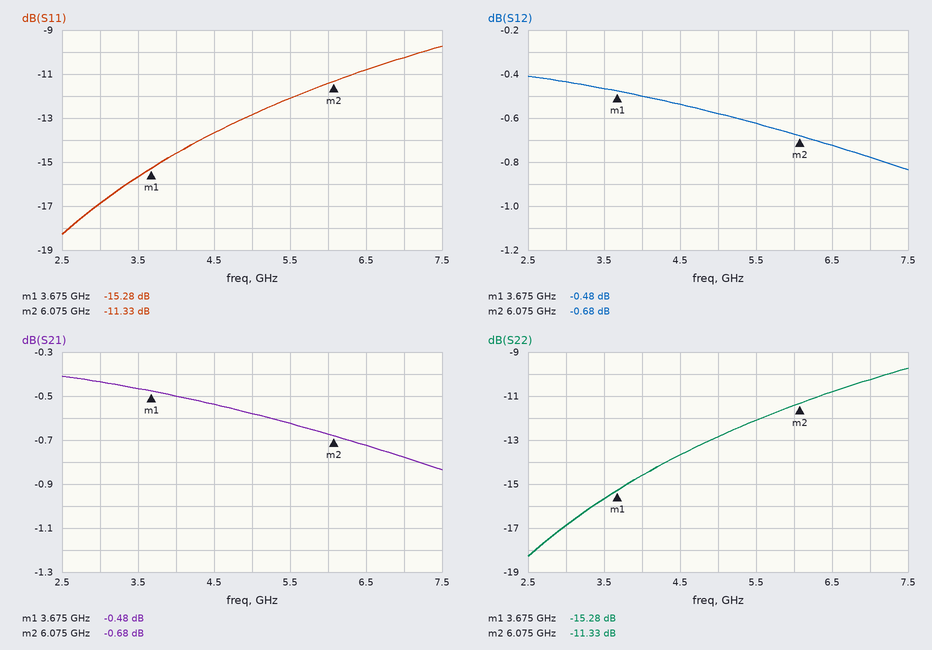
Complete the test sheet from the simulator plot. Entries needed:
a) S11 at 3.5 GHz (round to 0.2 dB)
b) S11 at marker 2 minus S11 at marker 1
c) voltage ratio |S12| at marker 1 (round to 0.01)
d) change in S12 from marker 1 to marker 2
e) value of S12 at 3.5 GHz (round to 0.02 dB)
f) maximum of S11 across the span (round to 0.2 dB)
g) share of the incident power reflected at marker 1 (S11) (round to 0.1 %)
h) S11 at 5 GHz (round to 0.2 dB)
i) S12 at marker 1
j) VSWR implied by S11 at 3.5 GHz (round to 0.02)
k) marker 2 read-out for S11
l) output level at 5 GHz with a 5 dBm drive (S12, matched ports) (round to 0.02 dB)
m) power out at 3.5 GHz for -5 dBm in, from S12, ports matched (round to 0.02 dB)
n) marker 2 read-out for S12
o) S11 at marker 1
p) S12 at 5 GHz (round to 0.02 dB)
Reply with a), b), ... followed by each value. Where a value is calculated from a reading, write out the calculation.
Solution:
a) -15.6 dB
b) -11.33 − (-15.28) = 3.95 dB
c) 10^(-0.48/20) ≈ 0.95
d) -0.68 − (-0.48) = -0.20 dB
e) -0.46 dB
f) -9.8 dB
g) 10^(-15.28/10) ≈ 3.0 %
h) -12.8 dB
i) -0.48 dB
j) |Γ| = 10^(-15.6/20) = 0.1660; VSWR = (1 + 0.1660)/(1 − 0.1660) ≈ 1.40
k) -11.33 dB
l) 5 dBm + (-0.58 dB) = 4.42 dBm
m) -5 dBm + (-0.46 dB) = -5.46 dBm
n) -0.68 dB
o) -15.28 dB
p) -0.58 dB
